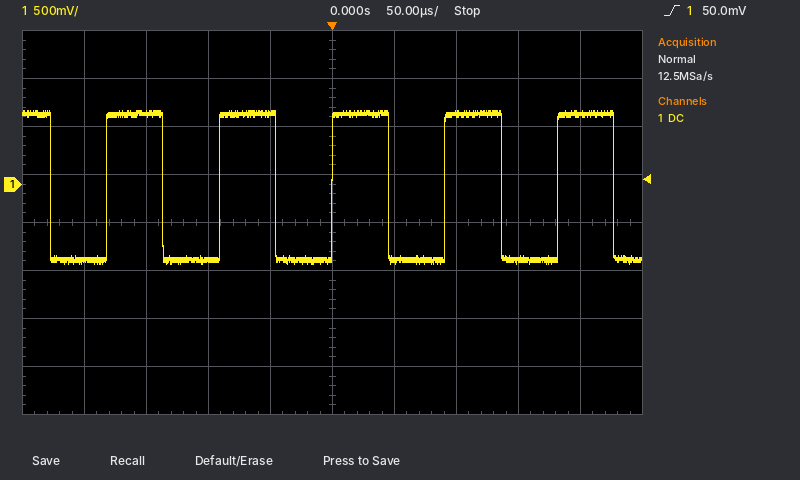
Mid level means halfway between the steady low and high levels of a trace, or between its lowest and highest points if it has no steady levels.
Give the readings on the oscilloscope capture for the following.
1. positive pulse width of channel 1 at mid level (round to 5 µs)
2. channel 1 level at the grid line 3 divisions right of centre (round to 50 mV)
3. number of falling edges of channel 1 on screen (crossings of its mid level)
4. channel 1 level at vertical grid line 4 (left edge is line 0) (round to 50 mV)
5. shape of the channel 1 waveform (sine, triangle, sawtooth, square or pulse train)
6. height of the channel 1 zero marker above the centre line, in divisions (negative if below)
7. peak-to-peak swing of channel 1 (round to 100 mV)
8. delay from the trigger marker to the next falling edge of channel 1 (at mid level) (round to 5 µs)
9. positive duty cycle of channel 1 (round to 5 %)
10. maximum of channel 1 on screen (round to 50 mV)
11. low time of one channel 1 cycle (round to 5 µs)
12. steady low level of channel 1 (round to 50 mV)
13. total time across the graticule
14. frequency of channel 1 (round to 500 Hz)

45 µs
-800 mV
6
750 mV
square
+0.8 div
1.60 V
45 µs
50 %
750 mV
45 µs
-800 mV
500 µs
11.0 kHz
